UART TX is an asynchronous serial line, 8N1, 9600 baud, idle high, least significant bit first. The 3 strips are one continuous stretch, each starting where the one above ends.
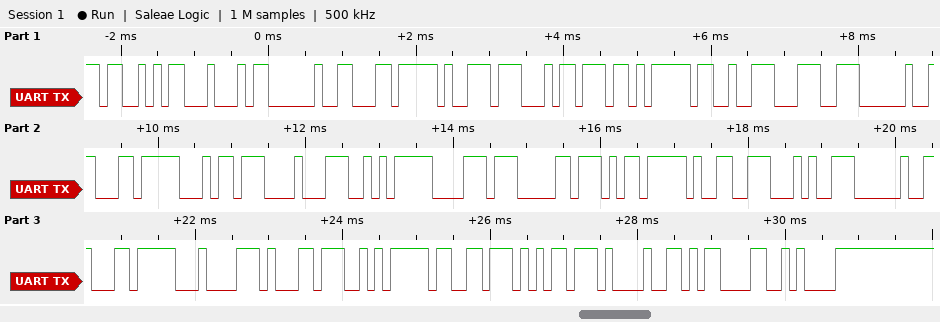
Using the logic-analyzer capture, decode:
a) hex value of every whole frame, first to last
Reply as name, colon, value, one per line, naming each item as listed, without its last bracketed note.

hex value of every whole frame, first to last: 53 44 20 EC B9 B4 EB 93 9C 20 EC B4 88 EA B8 B0 ED 99 94 20 EC 84 B1 EA B3 B5 21 0D 0A
